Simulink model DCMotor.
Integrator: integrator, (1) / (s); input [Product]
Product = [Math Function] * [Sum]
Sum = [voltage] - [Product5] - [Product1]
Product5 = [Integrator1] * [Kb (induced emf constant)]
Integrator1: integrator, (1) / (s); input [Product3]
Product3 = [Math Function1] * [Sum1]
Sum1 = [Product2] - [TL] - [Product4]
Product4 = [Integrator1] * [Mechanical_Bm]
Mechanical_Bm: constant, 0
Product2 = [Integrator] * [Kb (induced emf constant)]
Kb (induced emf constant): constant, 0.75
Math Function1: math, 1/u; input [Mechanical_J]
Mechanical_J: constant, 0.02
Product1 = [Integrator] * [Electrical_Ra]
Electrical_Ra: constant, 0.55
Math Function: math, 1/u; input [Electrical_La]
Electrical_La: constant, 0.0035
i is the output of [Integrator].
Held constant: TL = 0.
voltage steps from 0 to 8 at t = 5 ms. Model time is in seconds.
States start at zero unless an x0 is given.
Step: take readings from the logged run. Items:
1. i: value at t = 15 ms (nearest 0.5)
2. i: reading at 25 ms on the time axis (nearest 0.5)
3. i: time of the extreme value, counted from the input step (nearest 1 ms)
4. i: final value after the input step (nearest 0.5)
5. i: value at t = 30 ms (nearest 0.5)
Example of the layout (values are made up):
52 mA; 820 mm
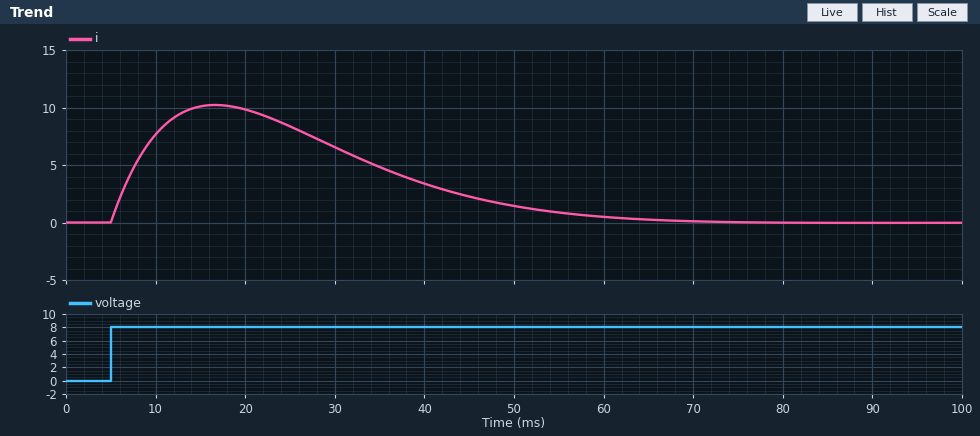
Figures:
10.0; 8.5; 12 ms; 0.0; 6.5
